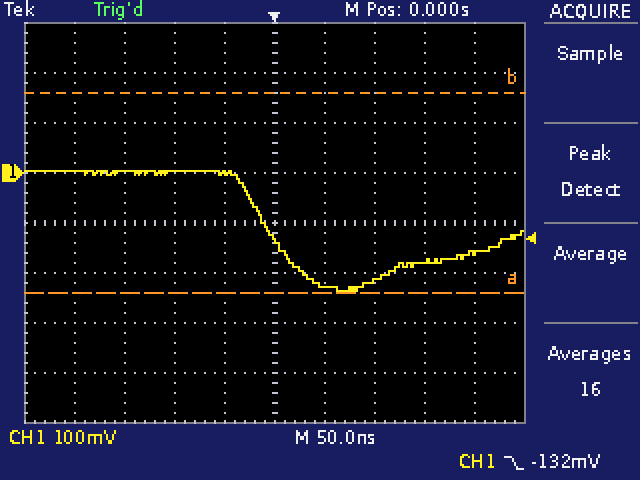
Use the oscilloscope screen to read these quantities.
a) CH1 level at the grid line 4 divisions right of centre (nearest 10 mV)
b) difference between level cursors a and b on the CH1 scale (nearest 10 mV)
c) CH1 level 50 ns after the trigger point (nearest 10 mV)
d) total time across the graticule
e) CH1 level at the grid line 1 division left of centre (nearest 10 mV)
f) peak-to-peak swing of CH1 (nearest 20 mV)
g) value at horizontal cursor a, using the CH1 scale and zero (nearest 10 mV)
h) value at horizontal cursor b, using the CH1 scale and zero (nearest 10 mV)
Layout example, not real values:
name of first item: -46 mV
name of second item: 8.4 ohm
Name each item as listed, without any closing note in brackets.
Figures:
CH1 level at the grid line 4 divisions right of centre: -160 mV
difference between level cursors a and b on the CH1 scale: 400 mV
CH1 level 50 ns after the trigger point: -230 mV
total time across the graticule: 500 ns
CH1 level at the grid line 1 division left of centre: 0 mV
peak-to-peak swing of CH1: 240 mV
value at horizontal cursor a, using the CH1 scale and zero: -240 mV
value at horizontal cursor b, using the CH1 scale and zero: 160 mV
